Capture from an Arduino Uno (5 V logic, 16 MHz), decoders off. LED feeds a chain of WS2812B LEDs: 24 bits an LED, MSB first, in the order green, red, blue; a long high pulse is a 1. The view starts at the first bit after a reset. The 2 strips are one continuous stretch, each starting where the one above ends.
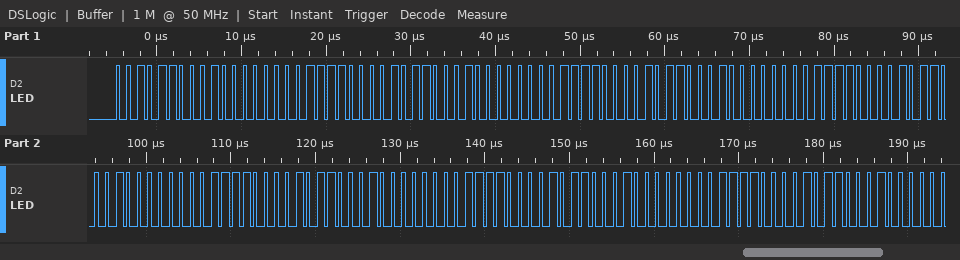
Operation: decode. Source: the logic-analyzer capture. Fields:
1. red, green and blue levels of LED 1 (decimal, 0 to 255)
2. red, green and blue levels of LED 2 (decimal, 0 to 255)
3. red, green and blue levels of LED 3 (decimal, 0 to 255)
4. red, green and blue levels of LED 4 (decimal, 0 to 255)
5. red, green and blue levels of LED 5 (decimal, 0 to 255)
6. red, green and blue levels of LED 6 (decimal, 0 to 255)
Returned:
64, 44, 60
64, 44, 60
64, 44, 60
64, 44, 60
64, 44, 60
64, 44, 60
